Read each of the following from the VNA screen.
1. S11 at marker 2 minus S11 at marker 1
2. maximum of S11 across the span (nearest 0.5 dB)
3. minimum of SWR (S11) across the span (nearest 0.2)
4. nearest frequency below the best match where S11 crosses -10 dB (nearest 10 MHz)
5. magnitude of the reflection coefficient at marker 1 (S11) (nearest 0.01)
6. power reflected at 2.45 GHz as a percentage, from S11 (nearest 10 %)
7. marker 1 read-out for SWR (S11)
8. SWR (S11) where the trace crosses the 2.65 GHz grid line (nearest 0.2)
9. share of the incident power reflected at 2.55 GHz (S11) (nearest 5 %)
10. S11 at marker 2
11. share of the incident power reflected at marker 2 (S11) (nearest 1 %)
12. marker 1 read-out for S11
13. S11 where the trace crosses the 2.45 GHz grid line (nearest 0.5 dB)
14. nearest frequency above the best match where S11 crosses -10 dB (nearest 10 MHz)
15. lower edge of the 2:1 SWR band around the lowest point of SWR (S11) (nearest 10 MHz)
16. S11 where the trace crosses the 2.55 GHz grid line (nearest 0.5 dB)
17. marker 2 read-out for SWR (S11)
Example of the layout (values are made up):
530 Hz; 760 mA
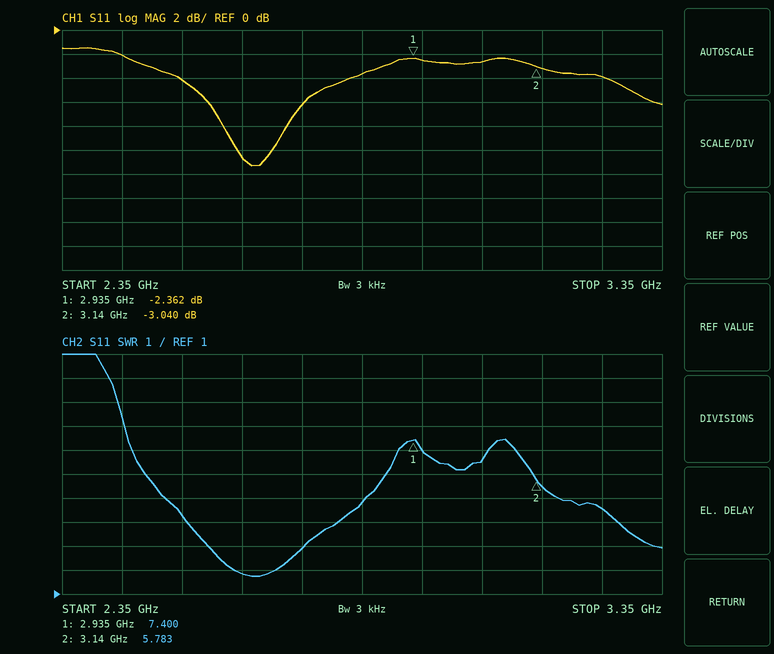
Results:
-0.678 dB; -1.5 dB; 1.8; 2.64 GHz; 0.76; 60 %; 7.400; 1.8; 40 %; -3.040 dB; 50 %; -2.362 dB; -2.0 dB; 2.70 GHz; 2.64 GHz; -4.0 dB; 5.783
